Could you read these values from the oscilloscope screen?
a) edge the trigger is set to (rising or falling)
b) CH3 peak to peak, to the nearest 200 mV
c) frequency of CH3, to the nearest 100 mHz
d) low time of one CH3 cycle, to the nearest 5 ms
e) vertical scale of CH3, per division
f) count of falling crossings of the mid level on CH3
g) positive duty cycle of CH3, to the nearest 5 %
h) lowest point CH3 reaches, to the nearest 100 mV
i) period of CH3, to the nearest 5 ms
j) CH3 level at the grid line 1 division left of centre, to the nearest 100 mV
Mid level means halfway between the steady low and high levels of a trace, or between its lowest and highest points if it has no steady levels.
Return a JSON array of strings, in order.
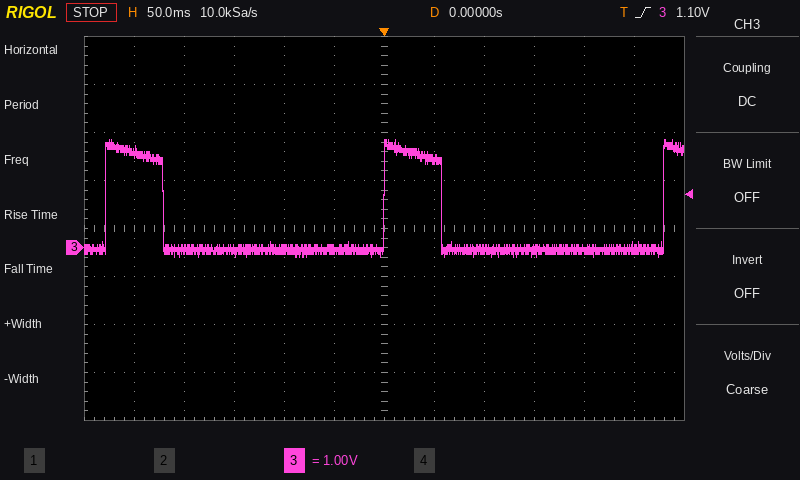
["rising", "2.4 V", "3.6 Hz", "220 ms", "1 V", "2", "20 %", "-200 mV", "280 ms", "0.0 V"]
